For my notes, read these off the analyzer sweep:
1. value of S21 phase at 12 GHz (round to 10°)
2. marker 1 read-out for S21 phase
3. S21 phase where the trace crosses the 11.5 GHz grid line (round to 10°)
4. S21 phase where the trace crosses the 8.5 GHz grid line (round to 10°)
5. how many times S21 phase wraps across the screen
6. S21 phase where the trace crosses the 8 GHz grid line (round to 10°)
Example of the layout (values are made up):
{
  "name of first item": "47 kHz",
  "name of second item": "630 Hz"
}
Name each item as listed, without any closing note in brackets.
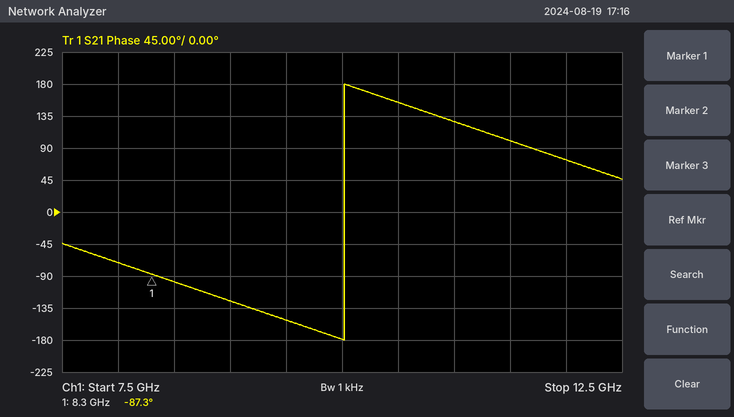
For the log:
{
  "value of S21 phase at 12 GHz": "70°",
  "marker 1 read-out for S21 phase": "-87.3°",
  "S21 phase where the trace crosses the 11.5 GHz grid line": "100°",
  "S21 phase where the trace crosses the 8.5 GHz grid line": "-100°",
  "how many times S21 phase wraps across the screen": "1",
  "S21 phase where the trace crosses the 8 GHz grid line": "-70°"
}
